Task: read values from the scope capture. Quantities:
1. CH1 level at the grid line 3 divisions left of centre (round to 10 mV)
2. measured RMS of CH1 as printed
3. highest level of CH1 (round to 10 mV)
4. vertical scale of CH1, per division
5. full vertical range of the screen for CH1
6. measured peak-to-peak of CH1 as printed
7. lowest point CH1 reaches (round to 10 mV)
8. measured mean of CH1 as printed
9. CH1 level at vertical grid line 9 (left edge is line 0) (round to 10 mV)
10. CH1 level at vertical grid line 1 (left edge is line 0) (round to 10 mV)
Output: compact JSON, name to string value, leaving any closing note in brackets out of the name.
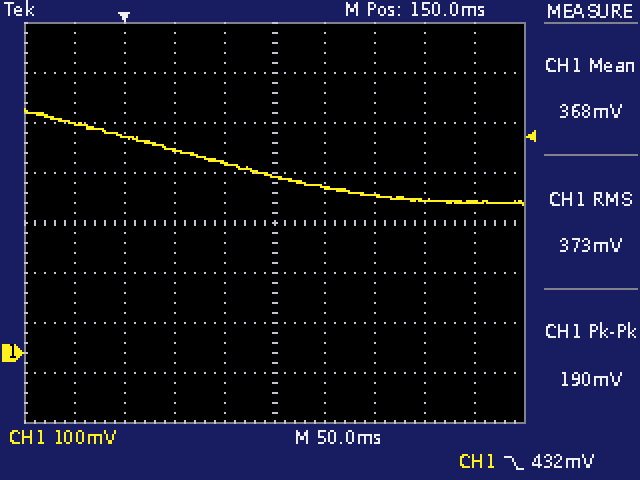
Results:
{"CH1 level at the grid line 3 divisions left of centre": "430 mV", "measured RMS of CH1 as printed": "373 mV", "highest level of CH1": "490 mV", "vertical scale of CH1, per division": "100 mV", "full vertical range of the screen for CH1": "800 mV", "measured peak-to-peak of CH1 as printed": "190 mV", "lowest point CH1 reaches": "300 mV", "measured mean of CH1 as printed": "368 mV", "CH1 level at vertical grid line 9 (left edge is line 0)": "300 mV", "CH1 level at vertical grid line 1 (left edge is line 0)": "460 mV"}
